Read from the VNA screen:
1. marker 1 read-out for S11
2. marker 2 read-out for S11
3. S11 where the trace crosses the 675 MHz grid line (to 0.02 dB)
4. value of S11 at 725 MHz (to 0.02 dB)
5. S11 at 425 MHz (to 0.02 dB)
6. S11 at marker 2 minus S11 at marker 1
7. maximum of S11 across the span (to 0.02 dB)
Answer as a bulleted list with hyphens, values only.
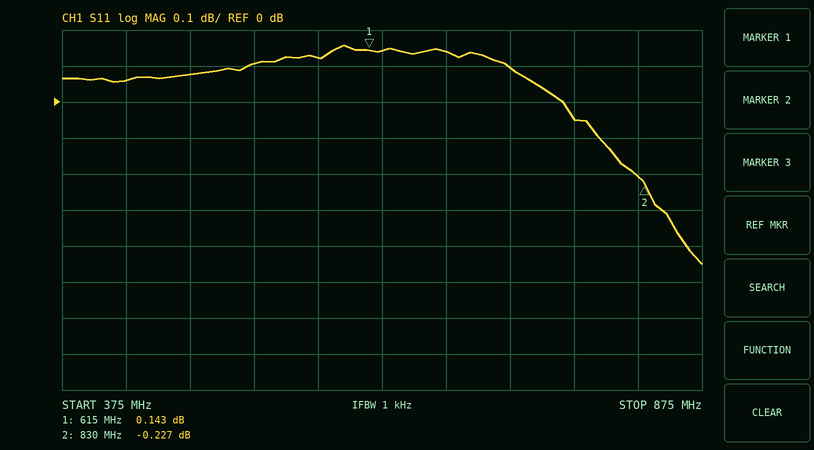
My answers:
- 0.143 dB
- -0.227 dB
- 0.14 dB
- 0.10 dB
- 0.06 dB
- -0.370 dB
- 0.16 dB
